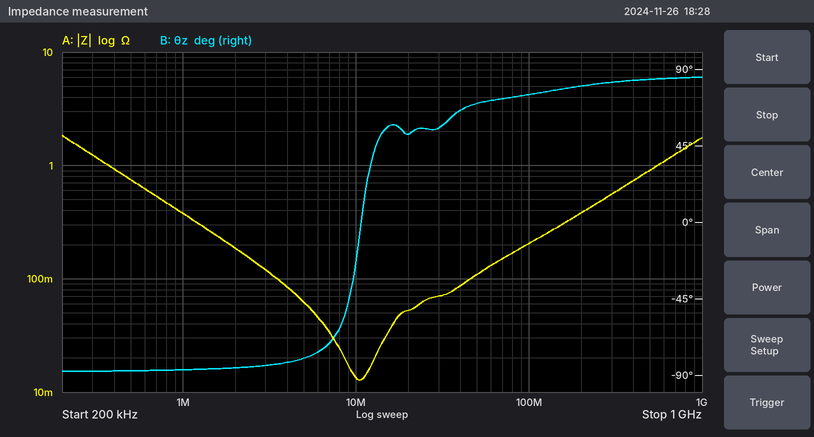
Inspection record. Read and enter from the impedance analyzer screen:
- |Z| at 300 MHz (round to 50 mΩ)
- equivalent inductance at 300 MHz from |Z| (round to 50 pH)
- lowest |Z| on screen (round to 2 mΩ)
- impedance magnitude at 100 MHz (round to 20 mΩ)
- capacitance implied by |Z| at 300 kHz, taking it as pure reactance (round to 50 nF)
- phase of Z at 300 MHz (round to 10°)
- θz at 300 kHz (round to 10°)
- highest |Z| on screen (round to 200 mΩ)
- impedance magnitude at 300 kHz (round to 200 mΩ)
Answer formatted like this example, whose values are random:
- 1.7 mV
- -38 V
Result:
- 550 mΩ
- 300 pH
- 12 mΩ
- 200 mΩ
- 450 nF
- 80°
- -90°
- 1.8 Ω
- 1.2 Ω
